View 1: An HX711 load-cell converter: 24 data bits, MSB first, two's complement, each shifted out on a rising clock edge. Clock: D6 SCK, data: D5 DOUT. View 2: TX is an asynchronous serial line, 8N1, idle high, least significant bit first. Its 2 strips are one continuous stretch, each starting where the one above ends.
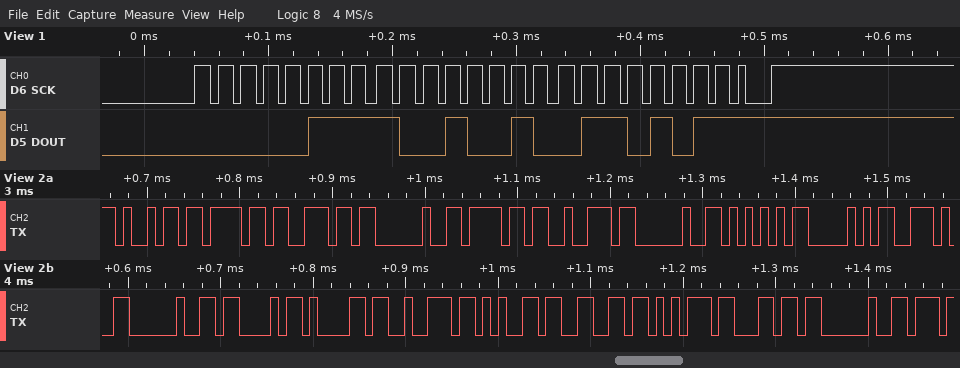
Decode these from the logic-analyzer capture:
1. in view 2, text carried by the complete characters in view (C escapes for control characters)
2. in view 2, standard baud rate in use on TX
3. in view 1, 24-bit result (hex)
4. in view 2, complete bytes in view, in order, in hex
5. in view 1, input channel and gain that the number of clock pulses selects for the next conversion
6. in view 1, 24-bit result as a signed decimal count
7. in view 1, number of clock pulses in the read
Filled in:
"ion or UP. Careful "
115200 baud
0x07926B
69 6F 6E 20 6F 72 20 55 50 2E 20 43 61 72 65 66 75 6C 20
channel B, gain 32
496235
26
